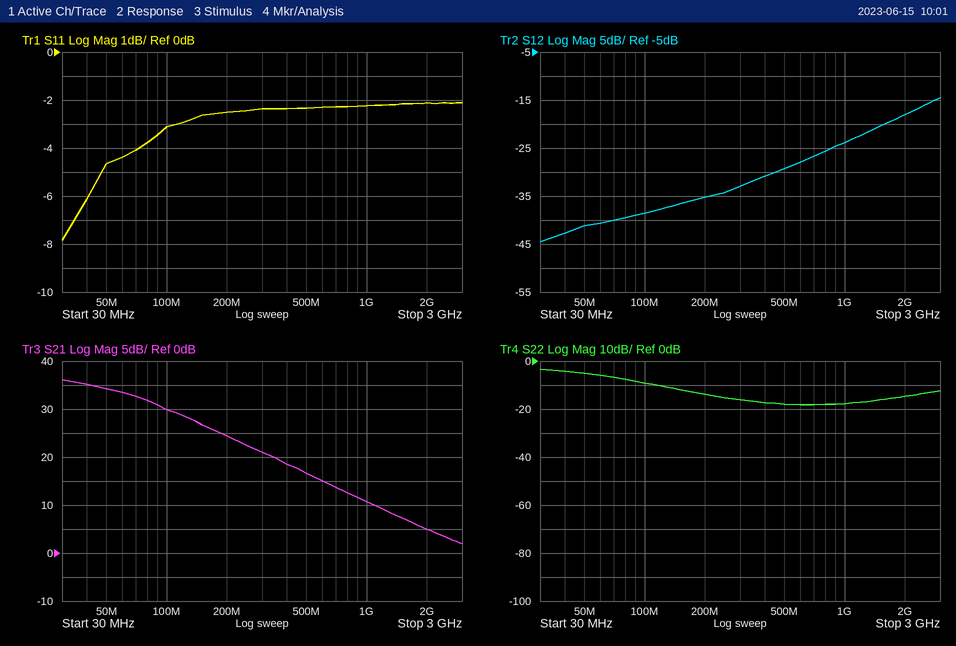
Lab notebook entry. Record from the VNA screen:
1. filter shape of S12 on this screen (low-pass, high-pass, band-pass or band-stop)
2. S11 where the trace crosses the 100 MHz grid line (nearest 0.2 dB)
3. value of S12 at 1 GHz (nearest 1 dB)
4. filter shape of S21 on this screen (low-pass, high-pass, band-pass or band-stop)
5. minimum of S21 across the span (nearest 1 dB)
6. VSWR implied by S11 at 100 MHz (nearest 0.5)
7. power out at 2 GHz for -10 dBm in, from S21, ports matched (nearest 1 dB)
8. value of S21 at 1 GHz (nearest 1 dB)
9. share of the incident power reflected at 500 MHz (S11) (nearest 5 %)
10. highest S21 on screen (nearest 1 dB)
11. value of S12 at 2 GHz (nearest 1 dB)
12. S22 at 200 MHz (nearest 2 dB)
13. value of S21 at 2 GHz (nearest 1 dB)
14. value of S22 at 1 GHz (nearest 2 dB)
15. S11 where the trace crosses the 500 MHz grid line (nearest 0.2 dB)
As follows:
high-pass
-3.2 dB
-24 dB
low-pass
2 dB
5.5
-5 dBm
11 dB
60 %
36 dB
-18 dB
-14 dB
5 dB
-18 dB
-2.4 dB
